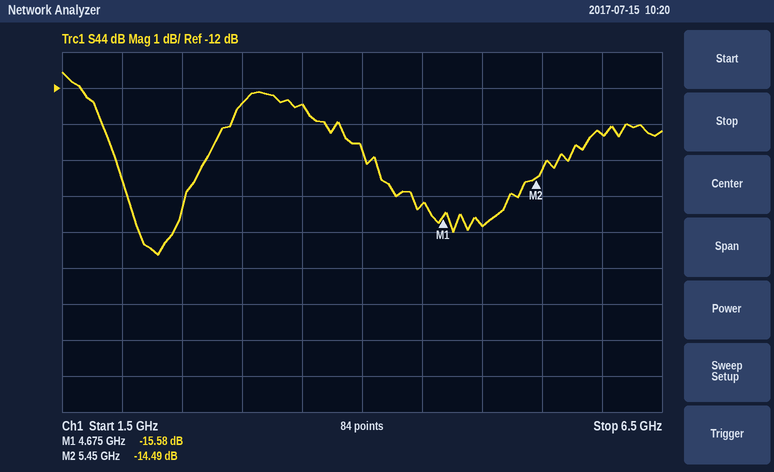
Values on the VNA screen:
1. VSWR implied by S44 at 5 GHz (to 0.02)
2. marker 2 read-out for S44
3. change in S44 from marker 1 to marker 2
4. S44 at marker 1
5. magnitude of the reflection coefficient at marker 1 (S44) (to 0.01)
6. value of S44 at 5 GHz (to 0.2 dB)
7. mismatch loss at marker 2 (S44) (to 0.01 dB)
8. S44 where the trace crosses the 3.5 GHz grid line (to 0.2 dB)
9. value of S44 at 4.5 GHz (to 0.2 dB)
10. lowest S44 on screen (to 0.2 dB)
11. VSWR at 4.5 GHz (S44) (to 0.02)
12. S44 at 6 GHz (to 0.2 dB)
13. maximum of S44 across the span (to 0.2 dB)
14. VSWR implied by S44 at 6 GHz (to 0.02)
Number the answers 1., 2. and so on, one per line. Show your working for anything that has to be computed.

1. |Γ| = 10^(-15.8/20) = 0.1622; VSWR = (1 + 0.1622)/(1 − 0.1622) ≈ 1.39, so 1.38 to the nearest 0.02
2. -14.49 dB
3. -14.49 − (-15.58) = 1.09 dB
4. -15.58 dB
5. 10^(-15.58/20) ≈ 0.17
6. -15.8 dB
7. −10 log10(1 − 10^(-14.49/10)) ≈ 0.16 dB
8. -12.4 dB
9. -15.2 dB
10. -16.6 dB
11. |Γ| = 10^(-15.2/20) = 0.1738; VSWR = (1 + 0.1738)/(1 − 0.1738) ≈ 1.42
12. -13.2 dB
13. -11.6 dB
14. |Γ| = 10^(-13.2/20) = 0.2188; VSWR = (1 + 0.2188)/(1 − 0.2188) ≈ 1.56
